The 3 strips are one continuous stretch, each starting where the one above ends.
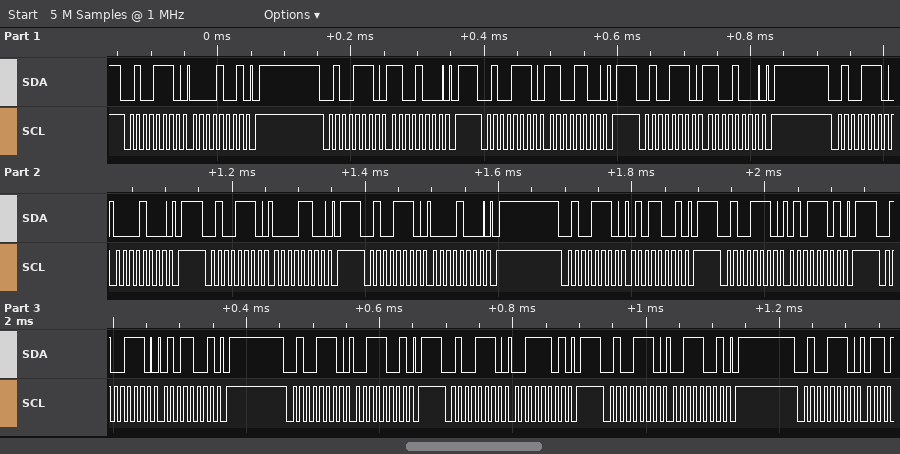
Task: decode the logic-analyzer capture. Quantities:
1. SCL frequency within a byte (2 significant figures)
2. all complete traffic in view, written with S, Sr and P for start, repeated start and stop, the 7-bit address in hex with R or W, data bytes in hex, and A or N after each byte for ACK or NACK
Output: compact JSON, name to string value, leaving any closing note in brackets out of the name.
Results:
{"SCL frequency within a byte": "100 kHz", "all complete traffic in view, written with S, Sr and P for start, repeated start and stop, the 7-bit address in hex with R or W, data bytes in hex, and A or N after each byte for ACK or NACK": "S 27W A 09 A P S 27W A C8 A P S 27W A CC A P S 27W A C8 A P S 27W A 08 A P S 27W A 0C A P S 27W A 08 A P S 27W A 59 A P S 27W A 5D A P S 27W A 59 A P S 27W A 39 A P S 27W A 3D A P S 27W A 39 A P S 27W A"}
